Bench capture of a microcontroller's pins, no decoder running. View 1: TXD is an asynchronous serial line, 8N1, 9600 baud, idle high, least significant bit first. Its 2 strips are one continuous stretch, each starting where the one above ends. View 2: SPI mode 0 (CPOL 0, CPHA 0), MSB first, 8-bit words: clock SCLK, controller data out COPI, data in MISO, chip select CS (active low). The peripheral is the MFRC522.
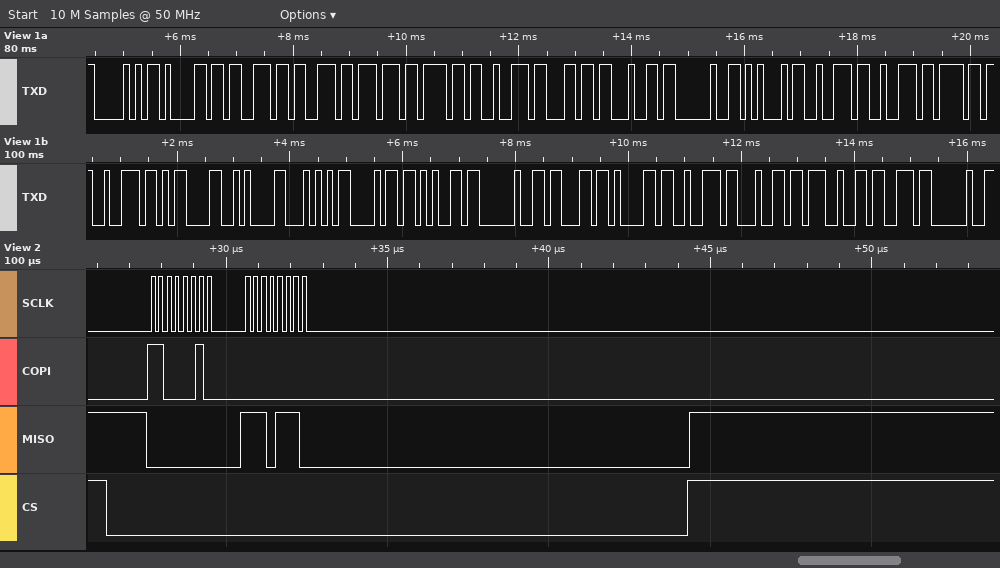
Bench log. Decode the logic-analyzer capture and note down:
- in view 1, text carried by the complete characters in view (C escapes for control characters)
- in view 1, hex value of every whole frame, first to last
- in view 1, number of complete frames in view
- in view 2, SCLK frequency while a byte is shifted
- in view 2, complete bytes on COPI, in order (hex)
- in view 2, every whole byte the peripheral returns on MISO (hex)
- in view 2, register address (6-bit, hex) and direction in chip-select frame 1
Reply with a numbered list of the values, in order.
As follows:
1. "Passworld Error\r\nThe card's "
2. 50 61 73 73 77 6F 72 6C 64 20 45 72 72 6F 72 0D 0A 54 68 65 20 63 61 72 64 27 73 20
3. 28
4. 4 MHz
5. C2 00
6. 00 EE
7. 0x21 read
